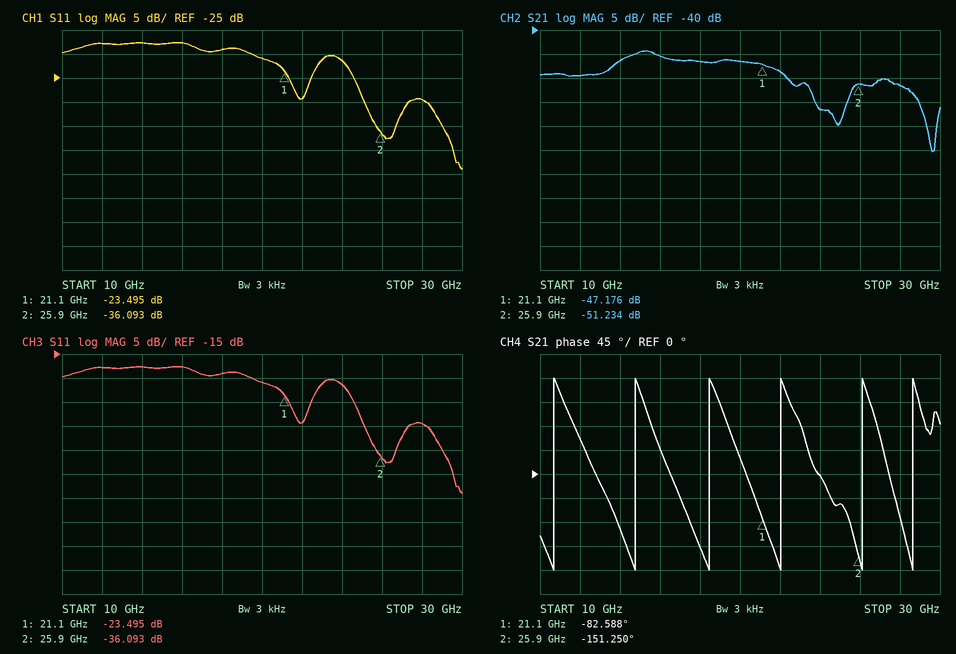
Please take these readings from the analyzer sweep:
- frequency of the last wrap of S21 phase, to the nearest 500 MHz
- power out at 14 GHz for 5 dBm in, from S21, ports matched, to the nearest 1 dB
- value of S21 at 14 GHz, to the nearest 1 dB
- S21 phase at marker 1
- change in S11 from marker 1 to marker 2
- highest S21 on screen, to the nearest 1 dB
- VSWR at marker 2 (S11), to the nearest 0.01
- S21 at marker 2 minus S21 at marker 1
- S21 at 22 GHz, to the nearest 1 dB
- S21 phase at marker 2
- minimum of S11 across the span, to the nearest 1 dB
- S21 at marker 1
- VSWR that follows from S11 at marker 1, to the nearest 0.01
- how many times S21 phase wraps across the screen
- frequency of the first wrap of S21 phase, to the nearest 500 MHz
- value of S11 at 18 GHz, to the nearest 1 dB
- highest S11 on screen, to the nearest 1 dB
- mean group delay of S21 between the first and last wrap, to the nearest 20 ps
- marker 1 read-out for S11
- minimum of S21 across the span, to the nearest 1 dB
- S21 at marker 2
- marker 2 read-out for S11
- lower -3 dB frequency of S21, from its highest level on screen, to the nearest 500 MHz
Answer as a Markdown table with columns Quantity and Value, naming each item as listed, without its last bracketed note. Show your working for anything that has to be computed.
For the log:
| Quantity | Value |
|---|---|
| frequency of the last wrap of S21 phase, to the nearest 500 MHz | 28.5 GHz |
| power out at 14 GHz for 5 dBm in, from S21, ports matched, to the nearest 1 dB | 5 dBm + (-46 dB) = -41 dBm |
| value of S21 at 14 GHz, to the nearest 1 dB | -46 dB |
| S21 phase at marker 1 | -82.588° |
| change in S11 from marker 1 to marker 2 | -36.093 − (-23.495) = -12.598 dB |
| highest S21 on screen, to the nearest 1 dB | -44 dB |
| VSWR at marker 2 (S11), to the nearest 0.01 | (1 + 0.0157)/(1 − 0.0157) ≈ 1.03 |
| S21 at marker 2 minus S21 at marker 1 | -51.234 − (-47.176) = -4.058 dB |
| S21 at 22 GHz, to the nearest 1 dB | -49 dB |
| S21 phase at marker 2 | -151.250° |
| minimum of S11 across the span, to the nearest 1 dB | -44 dB |
| S21 at marker 1 | -47.176 dB |
| VSWR that follows from S11 at marker 1, to the nearest 0.01 | (1 + 0.0669)/(1 − 0.0669) ≈ 1.14 |
| how many times S21 phase wraps across the screen | 6 |
| frequency of the first wrap of S21 phase, to the nearest 500 MHz | 10.5 GHz |
| value of S11 at 18 GHz, to the nearest 1 dB | -19 dB |
| highest S11 on screen, to the nearest 1 dB | -18 dB |
| mean group delay of S21 between the first and last wrap, to the nearest 20 ps | 5 cycles / (28.5 GHz − 10.5 GHz) ≈ 278 ps, so 280 ps to the nearest 20 ps |
| marker 1 read-out for S11 | -23.495 dB |
| minimum of S21 across the span, to the nearest 1 dB | -65 dB |
| S21 at marker 2 | -51.234 dB |
| marker 2 read-out for S11 | -36.093 dB |
| lower -3 dB frequency of S21, from its highest level on screen, to the nearest 500 MHz | 13.5 GHz |
